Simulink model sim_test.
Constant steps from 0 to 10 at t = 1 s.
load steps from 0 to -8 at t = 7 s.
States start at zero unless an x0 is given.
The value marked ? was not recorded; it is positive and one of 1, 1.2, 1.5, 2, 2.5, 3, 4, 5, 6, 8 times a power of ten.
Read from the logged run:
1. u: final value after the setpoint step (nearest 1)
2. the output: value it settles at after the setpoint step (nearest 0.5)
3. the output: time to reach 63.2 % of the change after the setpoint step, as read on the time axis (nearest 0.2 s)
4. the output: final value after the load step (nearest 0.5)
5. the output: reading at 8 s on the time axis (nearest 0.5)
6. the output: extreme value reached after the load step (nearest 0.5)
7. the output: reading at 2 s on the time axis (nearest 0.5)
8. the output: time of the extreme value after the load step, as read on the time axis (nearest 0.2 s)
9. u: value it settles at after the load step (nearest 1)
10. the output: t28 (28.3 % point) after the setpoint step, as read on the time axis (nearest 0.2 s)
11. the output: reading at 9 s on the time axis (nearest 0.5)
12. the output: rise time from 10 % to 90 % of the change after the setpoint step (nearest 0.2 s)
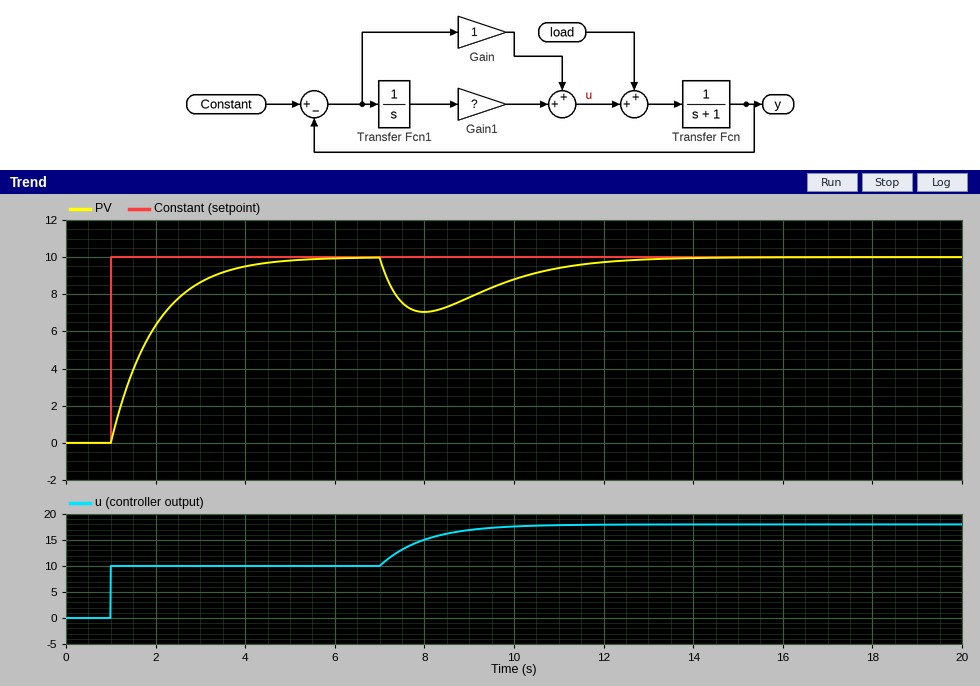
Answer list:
10
10.0
2.0 s
10.0
7.0
7.0
6.5
8.0 s
18
1.4 s
8.0
2.2 s
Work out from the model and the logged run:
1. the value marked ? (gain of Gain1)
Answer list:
1
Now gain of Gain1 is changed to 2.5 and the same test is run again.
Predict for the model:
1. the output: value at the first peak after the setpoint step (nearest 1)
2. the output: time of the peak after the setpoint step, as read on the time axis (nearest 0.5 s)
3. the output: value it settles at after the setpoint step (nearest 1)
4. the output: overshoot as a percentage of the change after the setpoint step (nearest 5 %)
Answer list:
11
3.0 s
10
10 %
